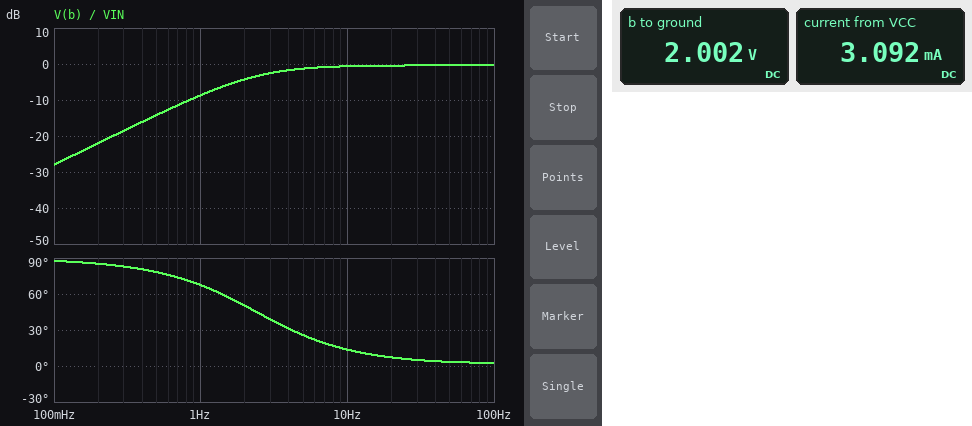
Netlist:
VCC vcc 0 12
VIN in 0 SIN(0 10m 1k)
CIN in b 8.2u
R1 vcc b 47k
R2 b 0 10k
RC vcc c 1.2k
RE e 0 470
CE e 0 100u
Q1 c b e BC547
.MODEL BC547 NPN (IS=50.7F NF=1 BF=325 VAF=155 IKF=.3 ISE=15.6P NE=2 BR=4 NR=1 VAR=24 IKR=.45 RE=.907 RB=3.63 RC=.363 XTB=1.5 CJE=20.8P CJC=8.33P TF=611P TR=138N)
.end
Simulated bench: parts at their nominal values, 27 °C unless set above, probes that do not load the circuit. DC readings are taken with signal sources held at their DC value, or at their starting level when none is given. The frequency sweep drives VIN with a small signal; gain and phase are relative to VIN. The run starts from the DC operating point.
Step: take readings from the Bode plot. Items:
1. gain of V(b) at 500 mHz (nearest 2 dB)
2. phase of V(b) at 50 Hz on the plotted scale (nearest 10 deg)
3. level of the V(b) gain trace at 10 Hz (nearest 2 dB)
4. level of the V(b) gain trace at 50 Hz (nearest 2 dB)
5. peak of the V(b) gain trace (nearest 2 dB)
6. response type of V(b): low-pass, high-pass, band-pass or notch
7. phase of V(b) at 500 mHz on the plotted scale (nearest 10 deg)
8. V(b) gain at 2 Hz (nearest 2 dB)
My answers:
-14 dB
0 deg
0 dB
0 dB
0 dB
high-pass
80 deg
-4 dB
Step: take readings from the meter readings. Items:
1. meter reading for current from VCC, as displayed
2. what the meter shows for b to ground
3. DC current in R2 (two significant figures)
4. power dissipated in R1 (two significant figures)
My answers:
3.092 mA
2.002 V
200 µA
2.1 mW
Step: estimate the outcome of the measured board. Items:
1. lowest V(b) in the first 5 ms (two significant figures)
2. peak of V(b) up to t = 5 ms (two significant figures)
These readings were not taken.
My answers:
2.0 V
2.0 V
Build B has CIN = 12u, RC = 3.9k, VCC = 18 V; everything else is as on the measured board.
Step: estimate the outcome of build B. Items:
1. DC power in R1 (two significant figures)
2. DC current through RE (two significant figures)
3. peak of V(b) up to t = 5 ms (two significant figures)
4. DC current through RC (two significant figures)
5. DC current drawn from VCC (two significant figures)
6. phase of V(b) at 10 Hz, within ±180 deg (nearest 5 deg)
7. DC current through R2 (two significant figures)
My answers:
5.0 mW
4.2 mA
2.6 V
4.1 mA
4.4 mA
30 deg
260 µA
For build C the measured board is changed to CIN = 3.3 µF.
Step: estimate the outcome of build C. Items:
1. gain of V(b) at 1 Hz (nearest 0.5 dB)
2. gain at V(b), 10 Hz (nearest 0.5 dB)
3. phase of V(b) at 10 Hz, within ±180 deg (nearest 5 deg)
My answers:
-16.0 dB
-2.0 dB
30 deg
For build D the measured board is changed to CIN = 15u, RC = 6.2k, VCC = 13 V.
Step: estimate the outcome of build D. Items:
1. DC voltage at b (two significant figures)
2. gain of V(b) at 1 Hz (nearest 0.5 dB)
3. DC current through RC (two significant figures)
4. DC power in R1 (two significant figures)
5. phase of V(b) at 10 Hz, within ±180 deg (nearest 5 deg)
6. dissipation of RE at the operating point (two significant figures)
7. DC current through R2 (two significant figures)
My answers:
1.6 V
-27.0 dB
1.9 mA
2.8 mW
35 deg
1.9 mW
160 µA
